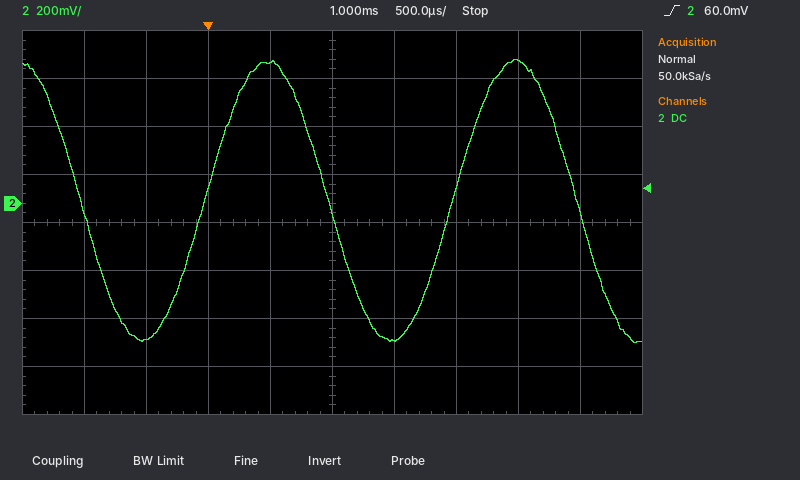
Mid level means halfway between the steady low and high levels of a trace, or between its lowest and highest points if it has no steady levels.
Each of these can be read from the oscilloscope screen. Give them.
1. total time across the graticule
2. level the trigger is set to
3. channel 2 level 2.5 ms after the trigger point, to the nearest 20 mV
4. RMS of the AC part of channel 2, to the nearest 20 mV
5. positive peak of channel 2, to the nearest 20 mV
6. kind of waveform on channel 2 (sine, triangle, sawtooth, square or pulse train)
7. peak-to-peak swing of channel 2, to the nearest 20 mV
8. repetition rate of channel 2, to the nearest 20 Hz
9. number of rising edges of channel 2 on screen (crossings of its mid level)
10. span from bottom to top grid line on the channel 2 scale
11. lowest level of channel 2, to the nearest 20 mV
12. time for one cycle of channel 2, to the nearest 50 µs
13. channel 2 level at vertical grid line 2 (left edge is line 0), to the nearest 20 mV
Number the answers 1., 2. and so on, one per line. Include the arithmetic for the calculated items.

1. 5 ms
2. 60.0 mV
3. 600 mV
4. 1.18 V / (2√2) ≈ 417 mV, so 420 mV to the nearest 20 mV
5. 600 mV
6. sine
7. 600 mV − (-580 mV) = 1.18 V
8. 1 / 2.00 ms ≈ 500 Hz
9. 2
10. 1.6 V
11. -580 mV
12. 2.00 ms
13. -560 mV
